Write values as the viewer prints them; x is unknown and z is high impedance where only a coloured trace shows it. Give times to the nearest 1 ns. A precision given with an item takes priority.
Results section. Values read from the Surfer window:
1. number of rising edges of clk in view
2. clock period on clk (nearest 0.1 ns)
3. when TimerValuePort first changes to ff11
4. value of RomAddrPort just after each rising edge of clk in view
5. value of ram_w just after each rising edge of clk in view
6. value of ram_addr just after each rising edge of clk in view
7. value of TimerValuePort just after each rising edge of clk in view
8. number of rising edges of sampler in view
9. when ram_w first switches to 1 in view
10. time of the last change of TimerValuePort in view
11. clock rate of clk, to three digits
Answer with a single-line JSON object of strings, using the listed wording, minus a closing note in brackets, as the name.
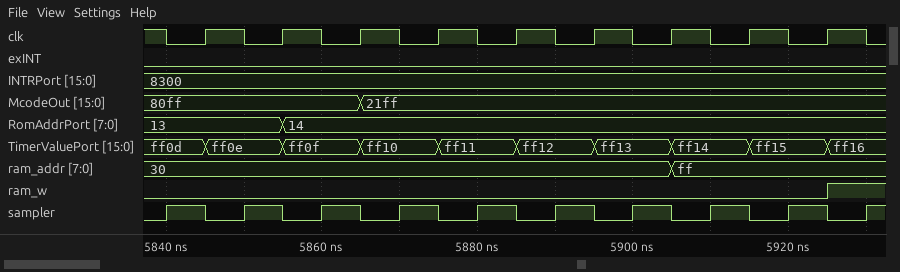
{"number of rising edges of clk in view": "9", "clock period on clk": "10 ns", "when TimerValuePort first changes to ff11": "5875 ns", "value of RomAddrPort just after each rising edge of clk in view": "13, 14, 14, 14, 14, 14, 14, 14, 14", "value of ram_w just after each rising edge of clk in view": "0 0 0 0 0 0 0 0 1", "value of ram_addr just after each rising edge of clk in view": "30, 30, 30, 30, 30, 30, ff, ff, ff", "value of TimerValuePort just after each rising edge of clk in view": "ff0e, ff0f, ff10, ff11, ff12, ff13, ff14, ff15, ff16", "number of rising edges of sampler in view": "10", "when ram_w first switches to 1 in view": "5925 ns", "time of the last change of TimerValuePort in view": "5925 ns", "clock rate of clk, to three digits": "100 MHz"}
